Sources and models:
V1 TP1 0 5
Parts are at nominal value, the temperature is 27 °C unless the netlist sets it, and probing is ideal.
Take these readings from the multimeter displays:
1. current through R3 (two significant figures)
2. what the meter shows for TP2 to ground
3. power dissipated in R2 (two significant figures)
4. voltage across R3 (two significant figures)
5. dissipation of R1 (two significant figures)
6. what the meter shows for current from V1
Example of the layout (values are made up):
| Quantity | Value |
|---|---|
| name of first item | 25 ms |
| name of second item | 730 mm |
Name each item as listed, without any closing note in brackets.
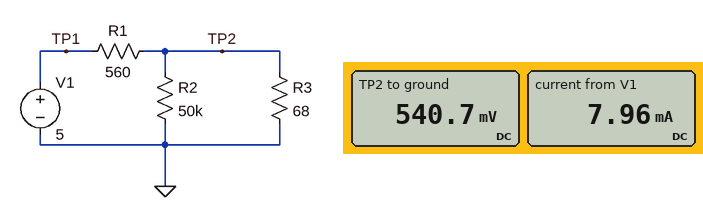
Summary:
| Quantity | Value |
|---|---|
| current through R3 | 8.0 mA |
| what the meter shows for TP2 to ground | 540.7 mV |
| power dissipated in R2 | 5.8 µW |
| voltage across R3 | 540 mV |
| dissipation of R1 | 36 mW |
| what the meter shows for current from V1 | 7.96 mA |
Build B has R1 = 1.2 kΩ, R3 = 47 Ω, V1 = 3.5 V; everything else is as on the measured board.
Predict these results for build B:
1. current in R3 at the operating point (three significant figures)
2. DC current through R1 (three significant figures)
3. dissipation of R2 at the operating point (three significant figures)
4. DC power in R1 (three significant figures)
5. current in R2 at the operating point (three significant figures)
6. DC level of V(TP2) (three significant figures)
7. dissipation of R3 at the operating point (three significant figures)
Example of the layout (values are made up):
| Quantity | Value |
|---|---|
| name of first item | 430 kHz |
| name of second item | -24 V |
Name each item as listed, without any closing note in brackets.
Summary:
| Quantity | Value |
|---|---|
| current in R3 at the operating point | 2.80 mA |
| DC current through R1 | 2.81 mA |
| dissipation of R2 at the operating point | 347 nW |
| DC power in R1 | 9.45 mW |
| current in R2 at the operating point | 2.64 µA |
| DC level of V(TP2) | 132 mV |
| dissipation of R3 at the operating point | 370 µW |
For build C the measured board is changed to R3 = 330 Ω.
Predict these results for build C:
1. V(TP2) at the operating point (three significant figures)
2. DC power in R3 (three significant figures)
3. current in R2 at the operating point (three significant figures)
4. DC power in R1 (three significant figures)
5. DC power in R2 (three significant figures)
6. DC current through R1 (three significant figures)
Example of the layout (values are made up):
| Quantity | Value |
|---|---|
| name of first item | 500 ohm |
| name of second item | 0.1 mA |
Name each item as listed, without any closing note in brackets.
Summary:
| Quantity | Value |
|---|---|
| V(TP2) at the operating point | 1.85 V |
| DC power in R3 | 10.3 mW |
| current in R2 at the operating point | 36.9 µA |
| DC power in R1 | 17.8 mW |
| DC power in R2 | 68.2 µW |
| DC current through R1 | 5.63 mA |
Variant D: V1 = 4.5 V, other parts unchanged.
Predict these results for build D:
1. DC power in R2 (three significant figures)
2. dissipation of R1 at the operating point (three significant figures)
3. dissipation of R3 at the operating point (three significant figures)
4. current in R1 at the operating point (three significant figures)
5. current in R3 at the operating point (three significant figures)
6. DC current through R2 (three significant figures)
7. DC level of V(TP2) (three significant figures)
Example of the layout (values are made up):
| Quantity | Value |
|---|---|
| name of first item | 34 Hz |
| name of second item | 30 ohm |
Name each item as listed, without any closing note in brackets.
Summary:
| Quantity | Value |
|---|---|
| DC power in R2 | 4.74 µW |
| dissipation of R1 at the operating point | 28.8 mW |
| dissipation of R3 at the operating point | 3.48 mW |
| current in R1 at the operating point | 7.17 mA |
| current in R3 at the operating point | 7.16 mA |
| DC current through R2 | 9.73 µA |
| DC level of V(TP2) | 487 mV |
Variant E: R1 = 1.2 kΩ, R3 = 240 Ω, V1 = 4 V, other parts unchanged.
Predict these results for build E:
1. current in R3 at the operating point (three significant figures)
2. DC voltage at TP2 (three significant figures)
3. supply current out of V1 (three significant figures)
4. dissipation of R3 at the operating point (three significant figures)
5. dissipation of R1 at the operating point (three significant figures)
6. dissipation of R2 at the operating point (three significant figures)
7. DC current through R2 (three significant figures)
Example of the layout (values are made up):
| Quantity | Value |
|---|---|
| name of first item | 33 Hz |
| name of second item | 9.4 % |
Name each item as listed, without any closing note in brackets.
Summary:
| Quantity | Value |
|---|---|
| current in R3 at the operating point | 2.77 mA |
| DC voltage at TP2 | 664 mV |
| supply current out of V1 | 2.78 mA |
| dissipation of R3 at the operating point | 1.84 mW |
| dissipation of R1 at the operating point | 9.27 mW |
| dissipation of R2 at the operating point | 8.82 µW |
| DC current through R2 | 13.3 µA |
